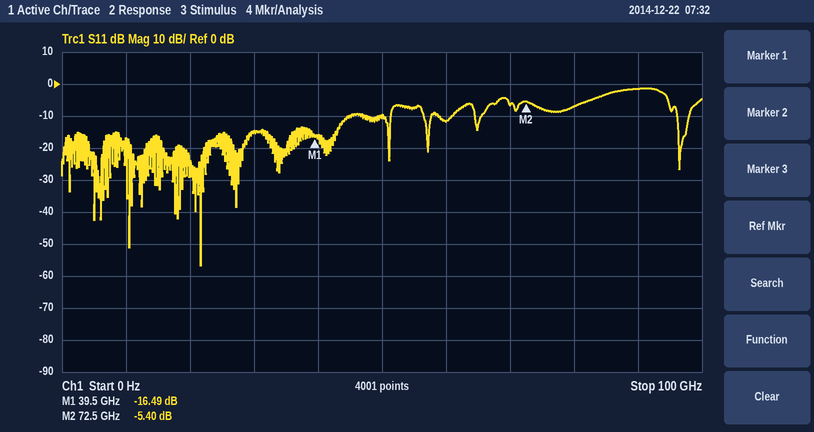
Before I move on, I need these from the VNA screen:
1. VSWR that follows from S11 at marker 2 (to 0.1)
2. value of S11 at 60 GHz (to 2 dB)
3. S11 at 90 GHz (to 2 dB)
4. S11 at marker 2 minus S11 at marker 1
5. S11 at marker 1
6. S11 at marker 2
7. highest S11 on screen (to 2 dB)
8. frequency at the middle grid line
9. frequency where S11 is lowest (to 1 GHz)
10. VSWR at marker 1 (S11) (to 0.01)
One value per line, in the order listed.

3.3
-12 dB
-2 dB
11.09 dB
-16.49 dB
-5.40 dB
-2 dB
50 GHz
22 GHz
1.35
